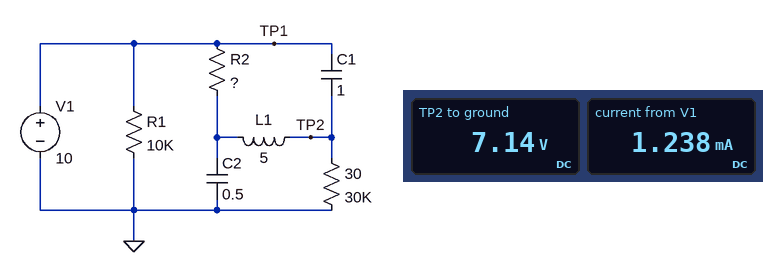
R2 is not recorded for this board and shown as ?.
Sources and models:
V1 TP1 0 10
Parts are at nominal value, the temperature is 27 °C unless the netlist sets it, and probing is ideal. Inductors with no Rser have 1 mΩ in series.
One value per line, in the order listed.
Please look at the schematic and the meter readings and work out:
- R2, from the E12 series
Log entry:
12 kΩ
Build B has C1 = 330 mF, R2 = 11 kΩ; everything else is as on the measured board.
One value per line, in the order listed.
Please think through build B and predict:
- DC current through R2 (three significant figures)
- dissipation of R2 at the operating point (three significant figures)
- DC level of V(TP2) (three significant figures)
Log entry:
244 µA
654 µW
7.32 V
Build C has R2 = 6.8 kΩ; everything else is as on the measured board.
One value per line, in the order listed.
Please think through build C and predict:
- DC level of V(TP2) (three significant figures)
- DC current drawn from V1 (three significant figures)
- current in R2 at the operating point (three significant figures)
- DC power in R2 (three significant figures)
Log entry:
8.15 V
1.27 mA
272 µA
502 µW
